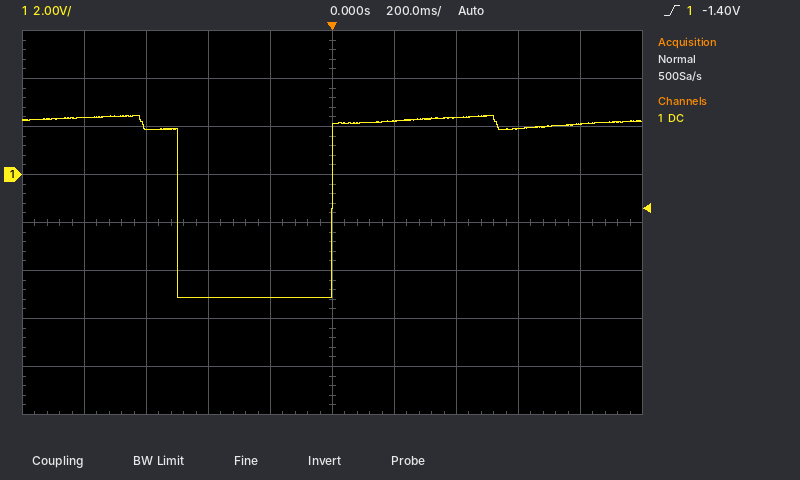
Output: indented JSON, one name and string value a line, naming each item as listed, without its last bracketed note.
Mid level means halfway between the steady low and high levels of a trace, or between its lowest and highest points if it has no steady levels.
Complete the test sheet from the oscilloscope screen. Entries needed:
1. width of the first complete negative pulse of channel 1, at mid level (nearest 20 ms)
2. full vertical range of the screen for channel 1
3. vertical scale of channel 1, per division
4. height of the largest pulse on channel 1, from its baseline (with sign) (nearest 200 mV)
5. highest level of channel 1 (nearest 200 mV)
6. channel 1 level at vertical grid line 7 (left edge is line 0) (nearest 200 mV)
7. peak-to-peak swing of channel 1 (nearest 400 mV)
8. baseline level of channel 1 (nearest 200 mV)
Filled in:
{
  "width of the first complete negative pulse of channel 1, at mid level": "500 ms",
  "full vertical range of the screen for channel 1": "16 V",
  "vertical scale of channel 1, per division": "2 V",
  "height of the largest pulse on channel 1, from its baseline (with sign)": "-7.4 V",
  "highest level of channel 1": "2.4 V",
  "channel 1 level at vertical grid line 7 (left edge is line 0)": "2.4 V",
  "peak-to-peak swing of channel 1": "7.6 V",
  "baseline level of channel 1": "2.2 V"
}
